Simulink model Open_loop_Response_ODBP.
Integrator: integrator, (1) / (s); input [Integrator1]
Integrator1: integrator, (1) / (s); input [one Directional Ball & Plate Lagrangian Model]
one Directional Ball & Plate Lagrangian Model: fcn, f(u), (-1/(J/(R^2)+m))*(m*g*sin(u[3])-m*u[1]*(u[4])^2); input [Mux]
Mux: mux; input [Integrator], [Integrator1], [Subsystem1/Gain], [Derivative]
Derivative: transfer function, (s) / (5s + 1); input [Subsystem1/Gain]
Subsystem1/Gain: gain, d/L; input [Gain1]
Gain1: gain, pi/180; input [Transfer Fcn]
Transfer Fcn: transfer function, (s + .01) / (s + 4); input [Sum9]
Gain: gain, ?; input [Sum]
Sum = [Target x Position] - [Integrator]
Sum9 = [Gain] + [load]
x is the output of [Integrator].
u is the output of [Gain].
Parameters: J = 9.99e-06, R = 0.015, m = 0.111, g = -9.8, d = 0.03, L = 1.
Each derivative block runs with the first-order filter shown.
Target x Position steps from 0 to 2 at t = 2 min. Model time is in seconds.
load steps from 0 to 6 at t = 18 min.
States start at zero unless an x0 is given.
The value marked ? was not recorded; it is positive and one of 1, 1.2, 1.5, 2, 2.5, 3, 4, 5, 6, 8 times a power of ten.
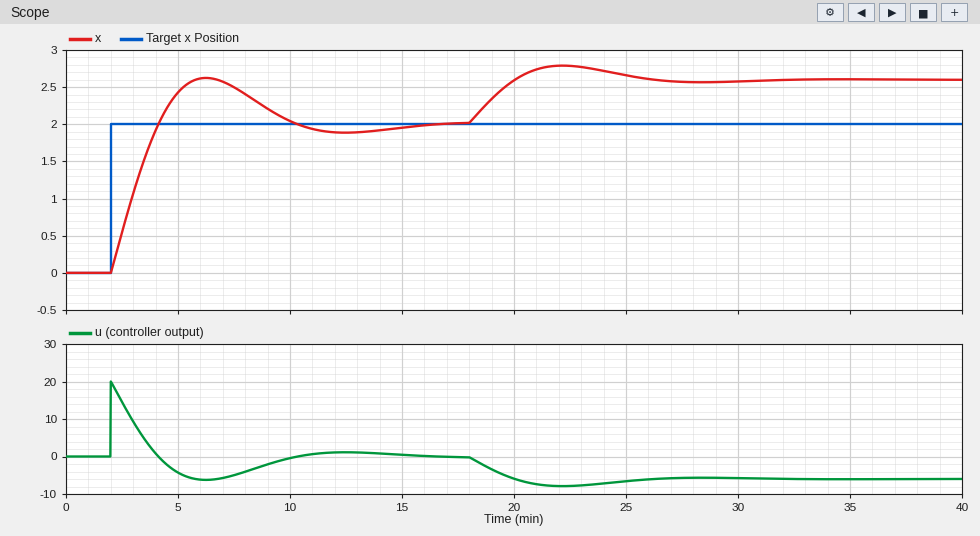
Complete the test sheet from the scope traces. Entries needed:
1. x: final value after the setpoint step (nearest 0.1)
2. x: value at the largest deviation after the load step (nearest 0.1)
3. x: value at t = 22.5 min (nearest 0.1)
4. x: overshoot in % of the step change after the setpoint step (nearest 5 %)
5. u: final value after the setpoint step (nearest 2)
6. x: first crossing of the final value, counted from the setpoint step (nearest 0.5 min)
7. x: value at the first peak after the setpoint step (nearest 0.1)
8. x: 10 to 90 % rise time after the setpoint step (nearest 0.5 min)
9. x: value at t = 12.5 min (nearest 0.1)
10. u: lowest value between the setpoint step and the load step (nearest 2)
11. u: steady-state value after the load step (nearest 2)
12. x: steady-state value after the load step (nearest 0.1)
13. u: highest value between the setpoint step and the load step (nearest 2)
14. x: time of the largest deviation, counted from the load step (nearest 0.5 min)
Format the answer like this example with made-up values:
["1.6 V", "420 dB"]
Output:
["2.0", "2.8", "2.8", "30 %", "0", "2.0 min", "2.6", "1.5 min", "1.9", "-6", "-6", "2.6", "20", "4.0 min"]
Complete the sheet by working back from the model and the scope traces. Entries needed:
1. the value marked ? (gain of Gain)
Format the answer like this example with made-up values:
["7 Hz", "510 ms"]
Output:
["10"]
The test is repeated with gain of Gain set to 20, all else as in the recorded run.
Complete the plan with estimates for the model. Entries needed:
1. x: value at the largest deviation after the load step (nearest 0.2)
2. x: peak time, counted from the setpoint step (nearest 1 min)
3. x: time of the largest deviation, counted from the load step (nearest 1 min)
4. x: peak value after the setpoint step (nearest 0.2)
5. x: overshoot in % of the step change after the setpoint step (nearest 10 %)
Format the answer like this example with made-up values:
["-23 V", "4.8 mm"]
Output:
["2.4", "3 min", "3 min", "2.4", "20 %"]
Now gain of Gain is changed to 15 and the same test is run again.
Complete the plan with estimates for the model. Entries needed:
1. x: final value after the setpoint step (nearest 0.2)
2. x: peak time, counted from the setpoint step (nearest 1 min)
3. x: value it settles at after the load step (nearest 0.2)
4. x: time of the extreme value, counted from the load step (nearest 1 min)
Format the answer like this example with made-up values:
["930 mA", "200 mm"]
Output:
["2.0", "3 min", "2.4", "3 min"]
